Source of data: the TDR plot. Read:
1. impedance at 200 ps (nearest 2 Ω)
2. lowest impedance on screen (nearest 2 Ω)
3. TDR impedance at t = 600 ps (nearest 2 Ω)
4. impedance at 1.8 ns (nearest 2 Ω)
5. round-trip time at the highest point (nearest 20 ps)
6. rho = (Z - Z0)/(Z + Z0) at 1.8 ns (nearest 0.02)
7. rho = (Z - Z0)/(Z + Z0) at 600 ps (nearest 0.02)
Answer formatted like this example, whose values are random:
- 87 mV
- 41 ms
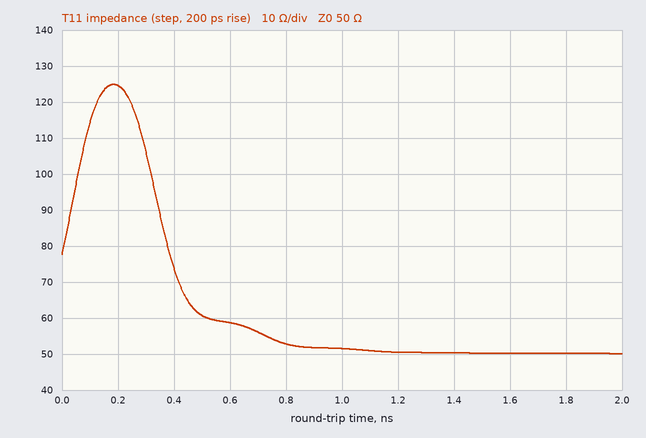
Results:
- 124 Ω
- 50 Ω
- 58 Ω
- 50 Ω
- 180 ps
- 0.00
- +0.08
